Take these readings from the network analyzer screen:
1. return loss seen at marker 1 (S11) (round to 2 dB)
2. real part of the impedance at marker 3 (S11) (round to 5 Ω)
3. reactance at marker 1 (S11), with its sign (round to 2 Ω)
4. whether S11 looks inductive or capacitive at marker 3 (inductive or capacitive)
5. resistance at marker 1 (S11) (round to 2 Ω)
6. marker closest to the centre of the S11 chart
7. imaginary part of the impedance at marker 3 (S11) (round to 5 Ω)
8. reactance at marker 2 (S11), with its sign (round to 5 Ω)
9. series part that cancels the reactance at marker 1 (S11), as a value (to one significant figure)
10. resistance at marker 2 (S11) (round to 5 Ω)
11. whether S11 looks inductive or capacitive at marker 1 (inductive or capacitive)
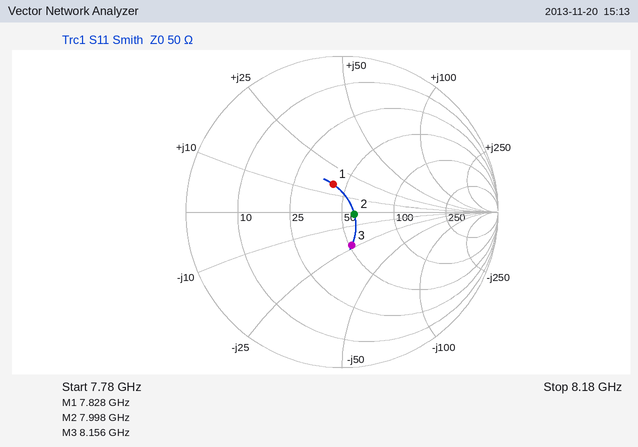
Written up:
14 dB
50 Ω
+16 Ω
capacitive
42 Ω
marker 2
-25 Ω
0 Ω
1 pF
60 Ω
inductive
